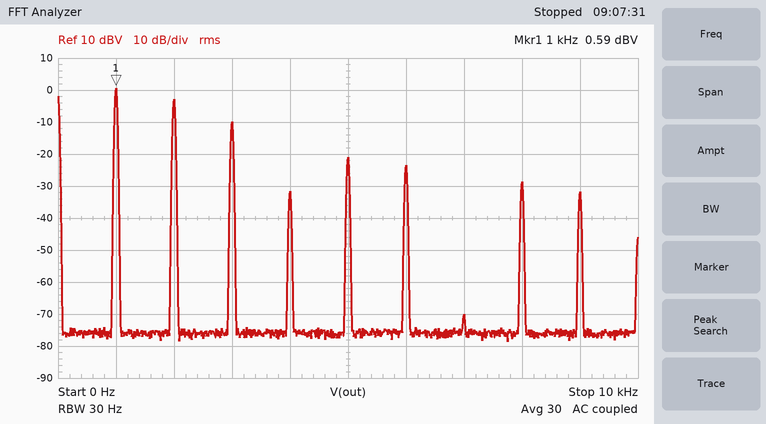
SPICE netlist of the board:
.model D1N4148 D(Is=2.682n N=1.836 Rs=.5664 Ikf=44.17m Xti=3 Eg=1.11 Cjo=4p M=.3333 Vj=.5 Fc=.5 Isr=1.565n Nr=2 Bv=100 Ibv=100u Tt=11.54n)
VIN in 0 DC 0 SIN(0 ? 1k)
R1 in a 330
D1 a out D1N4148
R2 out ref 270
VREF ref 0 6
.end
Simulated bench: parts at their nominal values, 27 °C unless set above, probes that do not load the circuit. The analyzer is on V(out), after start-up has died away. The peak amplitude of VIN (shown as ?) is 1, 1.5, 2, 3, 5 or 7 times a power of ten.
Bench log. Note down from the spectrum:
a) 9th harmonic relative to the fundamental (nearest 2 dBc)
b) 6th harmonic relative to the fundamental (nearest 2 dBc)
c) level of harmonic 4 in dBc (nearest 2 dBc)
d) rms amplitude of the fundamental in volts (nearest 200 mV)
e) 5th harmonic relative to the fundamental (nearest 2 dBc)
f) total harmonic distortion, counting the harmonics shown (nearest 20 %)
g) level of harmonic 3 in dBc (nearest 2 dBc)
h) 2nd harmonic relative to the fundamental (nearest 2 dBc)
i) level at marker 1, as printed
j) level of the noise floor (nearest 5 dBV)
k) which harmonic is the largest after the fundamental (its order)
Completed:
-32 dBc
-24 dBc
-32 dBc
1.0 V
-22 dBc
80 %
-10 dBc
-4 dBc
0.59 dBV
-75 dBV
2
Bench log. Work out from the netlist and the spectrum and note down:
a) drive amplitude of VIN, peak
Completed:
15 V
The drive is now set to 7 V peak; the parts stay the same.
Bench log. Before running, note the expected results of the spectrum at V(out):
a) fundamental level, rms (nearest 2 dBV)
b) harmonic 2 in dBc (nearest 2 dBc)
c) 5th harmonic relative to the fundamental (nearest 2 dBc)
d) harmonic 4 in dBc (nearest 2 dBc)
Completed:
-34 dBV
0 dBc
-4 dBc
-2 dBc
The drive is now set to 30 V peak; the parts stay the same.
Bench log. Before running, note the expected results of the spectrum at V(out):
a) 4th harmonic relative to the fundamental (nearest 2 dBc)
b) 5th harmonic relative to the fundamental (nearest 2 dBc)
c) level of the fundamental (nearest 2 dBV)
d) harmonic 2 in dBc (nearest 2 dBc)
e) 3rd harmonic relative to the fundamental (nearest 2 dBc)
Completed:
-22 dBc
-24 dBc
10 dBV
-6 dBc
-18 dBc
